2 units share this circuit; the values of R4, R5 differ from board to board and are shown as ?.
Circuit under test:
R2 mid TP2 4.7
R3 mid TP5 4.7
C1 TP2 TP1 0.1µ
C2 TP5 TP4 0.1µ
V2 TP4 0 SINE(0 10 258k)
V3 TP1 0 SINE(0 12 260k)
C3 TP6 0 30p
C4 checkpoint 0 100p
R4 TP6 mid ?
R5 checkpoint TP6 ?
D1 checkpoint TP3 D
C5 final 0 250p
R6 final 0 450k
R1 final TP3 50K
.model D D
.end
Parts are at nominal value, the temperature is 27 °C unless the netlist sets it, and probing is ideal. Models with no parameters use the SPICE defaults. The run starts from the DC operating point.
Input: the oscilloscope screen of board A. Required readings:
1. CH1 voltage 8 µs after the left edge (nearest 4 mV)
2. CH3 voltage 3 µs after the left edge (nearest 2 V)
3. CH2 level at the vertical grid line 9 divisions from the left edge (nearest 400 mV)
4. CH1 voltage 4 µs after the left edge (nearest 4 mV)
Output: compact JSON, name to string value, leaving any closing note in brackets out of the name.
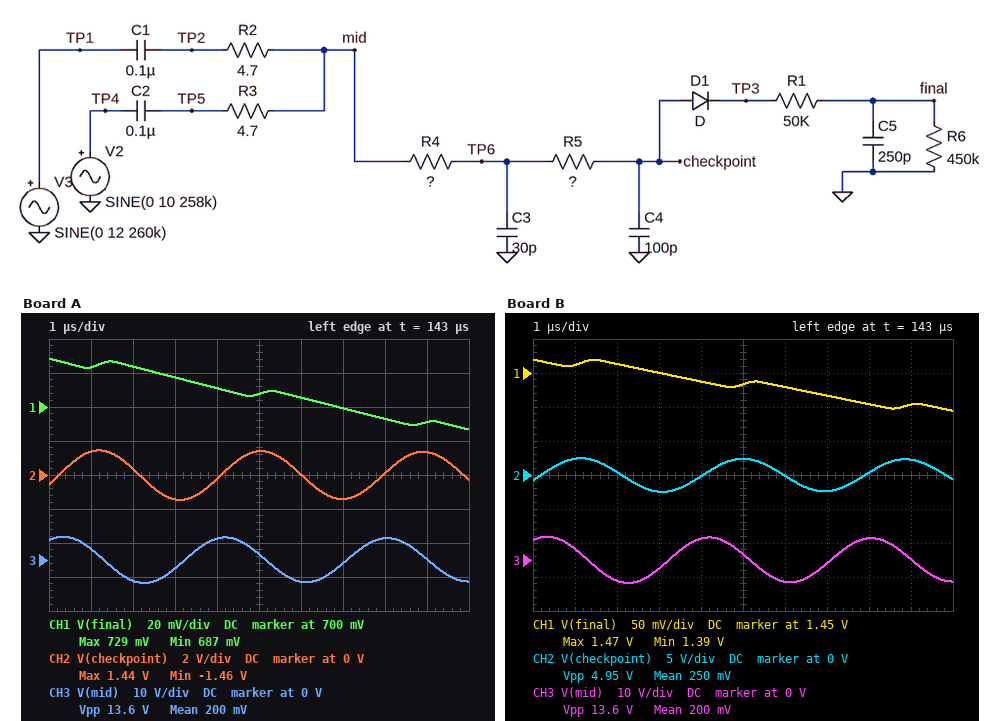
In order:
{"CH1 voltage 8 µs after the left edge": "692 mV", "CH3 voltage 3 µs after the left edge": "-2 V", "CH2 level at the vertical grid line 9 divisions from the left edge": "1.2 V", "CH1 voltage 4 µs after the left edge": "712 mV"}
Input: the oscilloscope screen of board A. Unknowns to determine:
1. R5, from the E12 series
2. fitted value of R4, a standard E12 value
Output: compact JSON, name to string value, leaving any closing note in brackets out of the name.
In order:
{"R5, from the E12 series": "27 kΩ", "fitted value of R4, a standard E12 value": "820 Ω"}
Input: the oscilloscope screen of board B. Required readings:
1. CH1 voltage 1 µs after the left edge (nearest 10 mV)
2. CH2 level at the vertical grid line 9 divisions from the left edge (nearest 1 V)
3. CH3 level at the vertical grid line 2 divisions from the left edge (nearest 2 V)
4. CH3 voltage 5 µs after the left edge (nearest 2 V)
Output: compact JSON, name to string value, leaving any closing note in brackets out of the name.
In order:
{"CH1 voltage 1 µs after the left edge": "1.46 V", "CH2 level at the vertical grid line 9 divisions from the left edge": "2 V", "CH3 level at the vertical grid line 2 divisions from the left edge": "-6 V", "CH3 voltage 5 µs after the left edge": "2 V"}
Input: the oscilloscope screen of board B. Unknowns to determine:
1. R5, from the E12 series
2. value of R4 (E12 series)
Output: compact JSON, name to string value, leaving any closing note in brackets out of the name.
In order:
{"R5, from the E12 series": "12 kΩ", "value of R4": "3.3 kΩ"}
